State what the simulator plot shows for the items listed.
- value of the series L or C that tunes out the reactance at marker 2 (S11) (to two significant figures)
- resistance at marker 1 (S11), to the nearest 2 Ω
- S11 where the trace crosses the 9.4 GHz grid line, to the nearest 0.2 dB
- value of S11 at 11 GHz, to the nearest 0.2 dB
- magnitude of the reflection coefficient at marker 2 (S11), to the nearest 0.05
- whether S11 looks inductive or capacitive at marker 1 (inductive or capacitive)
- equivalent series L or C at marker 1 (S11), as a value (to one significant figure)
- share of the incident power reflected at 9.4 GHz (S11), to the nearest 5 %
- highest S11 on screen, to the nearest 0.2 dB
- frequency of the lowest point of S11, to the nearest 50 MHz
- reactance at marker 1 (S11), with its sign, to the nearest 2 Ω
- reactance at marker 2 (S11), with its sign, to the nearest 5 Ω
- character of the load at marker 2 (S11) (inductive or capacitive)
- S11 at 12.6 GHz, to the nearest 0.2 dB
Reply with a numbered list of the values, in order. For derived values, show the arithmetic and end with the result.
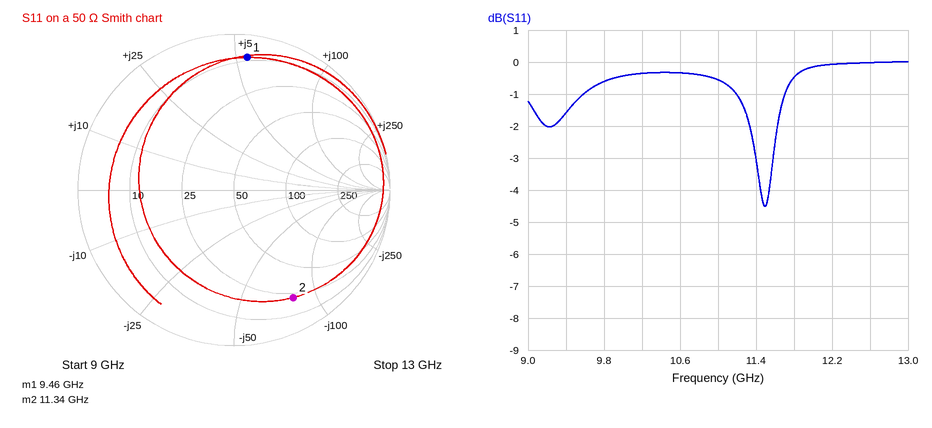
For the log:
1. L = 80 Ω/(2π × 11.34 GHz) ≈ 1.1 nH
2. 8 Ω
3. -1.6 dB
4. -0.6 dB
5. 0.80
6. inductive
7. L = 54 Ω/(2π × 9.46 GHz) ≈ 908 pH, so 900 pH to one significant figure
8. 10^(-1.6/10) ≈ 69.2 %, so 70 % to the nearest 5 %
9. 0.0 dB
10. 11.50 GHz
11. +54 Ω
12. -80 Ω
13. capacitive
14. 0.0 dB
